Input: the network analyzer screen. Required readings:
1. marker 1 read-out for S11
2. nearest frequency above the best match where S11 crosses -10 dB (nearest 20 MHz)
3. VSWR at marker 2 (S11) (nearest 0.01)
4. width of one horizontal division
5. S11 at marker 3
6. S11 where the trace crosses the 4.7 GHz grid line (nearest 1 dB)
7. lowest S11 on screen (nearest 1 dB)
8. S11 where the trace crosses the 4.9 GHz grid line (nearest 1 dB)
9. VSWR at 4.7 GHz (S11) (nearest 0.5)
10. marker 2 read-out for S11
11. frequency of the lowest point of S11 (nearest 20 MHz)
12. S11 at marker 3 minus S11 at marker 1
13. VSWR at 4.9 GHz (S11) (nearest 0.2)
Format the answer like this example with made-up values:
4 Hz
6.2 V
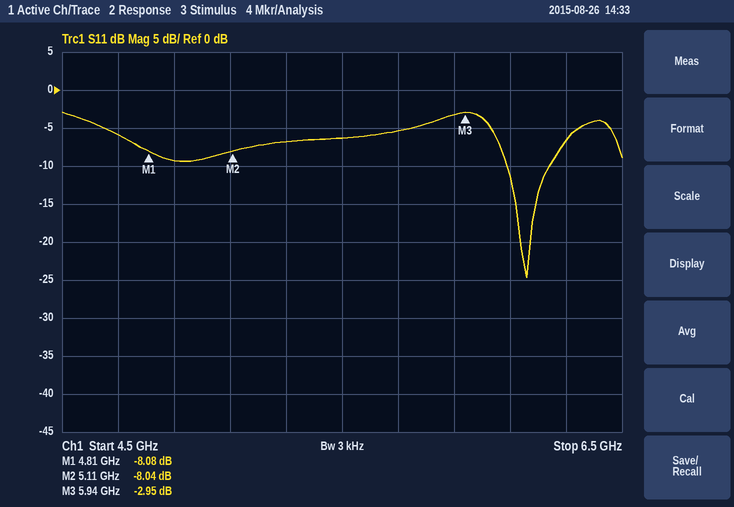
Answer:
-8.08 dB
6.24 GHz
2.31
200 MHz
-2.95 dB
-6 dB
-25 dB
-9 dB
3.0
-8.04 dB
6.16 GHz
5.13 dB
2.0
